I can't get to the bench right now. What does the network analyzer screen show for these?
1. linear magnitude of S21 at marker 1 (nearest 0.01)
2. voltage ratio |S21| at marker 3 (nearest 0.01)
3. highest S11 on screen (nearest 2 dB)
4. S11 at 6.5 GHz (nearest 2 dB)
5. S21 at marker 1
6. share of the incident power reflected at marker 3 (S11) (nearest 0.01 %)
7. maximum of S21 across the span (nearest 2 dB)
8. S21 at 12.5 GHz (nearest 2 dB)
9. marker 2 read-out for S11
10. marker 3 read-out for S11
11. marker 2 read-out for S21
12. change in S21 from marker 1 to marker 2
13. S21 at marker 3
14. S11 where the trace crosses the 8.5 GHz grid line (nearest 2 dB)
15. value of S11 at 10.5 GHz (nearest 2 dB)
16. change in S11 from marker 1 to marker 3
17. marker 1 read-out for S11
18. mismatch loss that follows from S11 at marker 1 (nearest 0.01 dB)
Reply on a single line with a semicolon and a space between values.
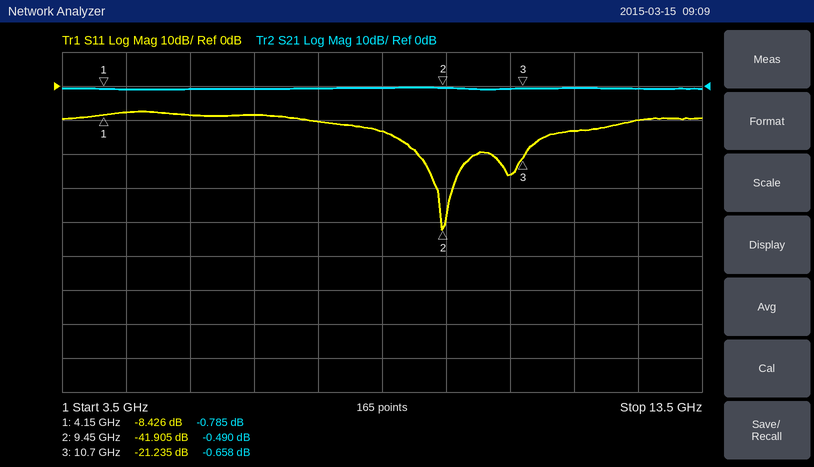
0.91; 0.93; -8 dB; -8 dB; -0.785 dB; 0.75 %; 0 dB; 0 dB; -41.905 dB; -21.235 dB; -0.490 dB; 0.295 dB; -0.658 dB; -14 dB; -26 dB; -12.809 dB; -8.426 dB; 0.67 dB
